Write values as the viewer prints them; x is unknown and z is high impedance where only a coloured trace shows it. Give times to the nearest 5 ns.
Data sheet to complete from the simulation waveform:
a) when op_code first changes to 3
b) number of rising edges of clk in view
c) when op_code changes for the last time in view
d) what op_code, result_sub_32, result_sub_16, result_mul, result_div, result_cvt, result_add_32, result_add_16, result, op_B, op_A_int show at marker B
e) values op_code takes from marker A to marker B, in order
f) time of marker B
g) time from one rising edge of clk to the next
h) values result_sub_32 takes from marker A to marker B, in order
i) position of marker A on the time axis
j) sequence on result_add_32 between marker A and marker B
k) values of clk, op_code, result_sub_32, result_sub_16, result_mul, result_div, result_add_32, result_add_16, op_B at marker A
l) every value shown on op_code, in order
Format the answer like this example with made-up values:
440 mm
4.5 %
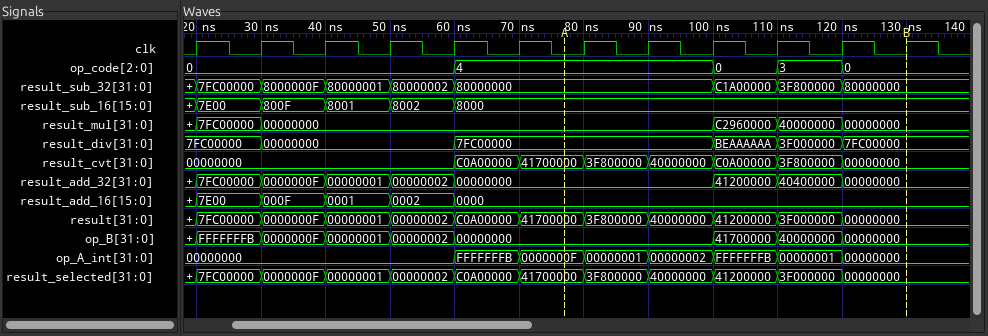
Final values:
110 ns
12
120 ns
op_code=0, result_sub_32=80000000, result_sub_16=8000, result_mul=00000000, result_div=7FC00000, result_cvt=00000000, result_add_32=00000000, result_add_16=0000, result=00000000, op_B=00000000, op_A_int=00000000
4, 0, 3, 0
130 ns
10 ns
80000000, C1A00000, 3F800000, 80000000
75 ns
00000000, 41200000, 40400000, 00000000
clk=0, op_code=4, result_sub_32=80000000, result_sub_16=8000, result_mul=00000000, result_div=7FC00000, result_add_32=00000000, result_add_16=0000, op_B=00000000
0, 4, 0, 3, 0
